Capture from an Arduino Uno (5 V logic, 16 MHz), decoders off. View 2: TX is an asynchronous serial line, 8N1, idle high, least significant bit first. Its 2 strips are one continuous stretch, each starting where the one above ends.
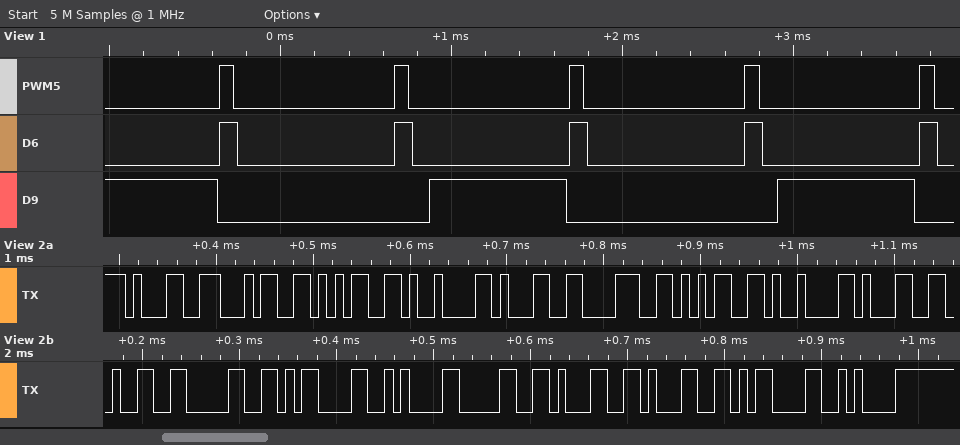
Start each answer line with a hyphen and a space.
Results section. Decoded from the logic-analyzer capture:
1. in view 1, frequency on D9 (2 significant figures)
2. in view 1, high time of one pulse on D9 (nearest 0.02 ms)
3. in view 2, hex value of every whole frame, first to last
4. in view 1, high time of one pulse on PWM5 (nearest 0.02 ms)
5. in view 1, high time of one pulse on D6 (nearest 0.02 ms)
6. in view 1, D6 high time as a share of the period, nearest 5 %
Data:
- 490 Hz
- 0.80 ms
- 0x31 0x34 0x35 0x09 0x31 0x38 0x35 0x09 0x31 0x32 0x30 0x0D 0x0A 0x30 0x31 0x31 0x0D 0x0A
- 0.08 ms
- 0.10 ms
- 10 %
